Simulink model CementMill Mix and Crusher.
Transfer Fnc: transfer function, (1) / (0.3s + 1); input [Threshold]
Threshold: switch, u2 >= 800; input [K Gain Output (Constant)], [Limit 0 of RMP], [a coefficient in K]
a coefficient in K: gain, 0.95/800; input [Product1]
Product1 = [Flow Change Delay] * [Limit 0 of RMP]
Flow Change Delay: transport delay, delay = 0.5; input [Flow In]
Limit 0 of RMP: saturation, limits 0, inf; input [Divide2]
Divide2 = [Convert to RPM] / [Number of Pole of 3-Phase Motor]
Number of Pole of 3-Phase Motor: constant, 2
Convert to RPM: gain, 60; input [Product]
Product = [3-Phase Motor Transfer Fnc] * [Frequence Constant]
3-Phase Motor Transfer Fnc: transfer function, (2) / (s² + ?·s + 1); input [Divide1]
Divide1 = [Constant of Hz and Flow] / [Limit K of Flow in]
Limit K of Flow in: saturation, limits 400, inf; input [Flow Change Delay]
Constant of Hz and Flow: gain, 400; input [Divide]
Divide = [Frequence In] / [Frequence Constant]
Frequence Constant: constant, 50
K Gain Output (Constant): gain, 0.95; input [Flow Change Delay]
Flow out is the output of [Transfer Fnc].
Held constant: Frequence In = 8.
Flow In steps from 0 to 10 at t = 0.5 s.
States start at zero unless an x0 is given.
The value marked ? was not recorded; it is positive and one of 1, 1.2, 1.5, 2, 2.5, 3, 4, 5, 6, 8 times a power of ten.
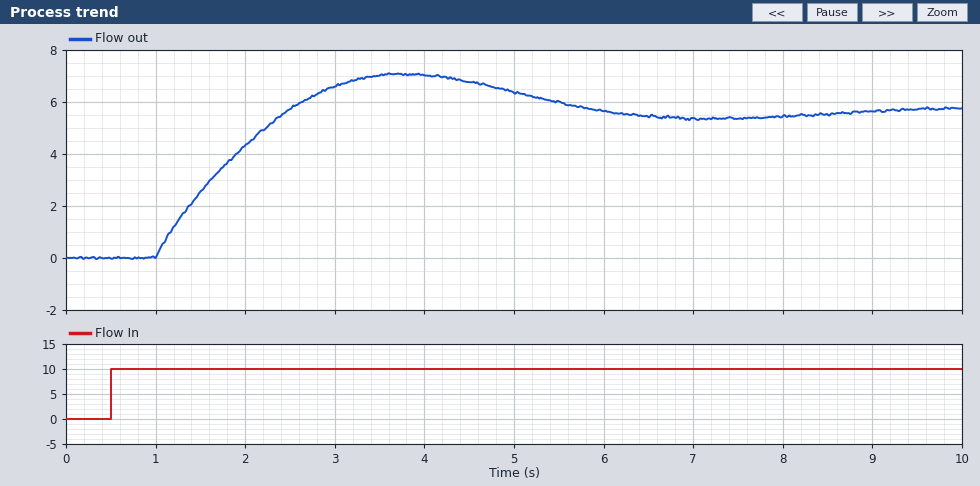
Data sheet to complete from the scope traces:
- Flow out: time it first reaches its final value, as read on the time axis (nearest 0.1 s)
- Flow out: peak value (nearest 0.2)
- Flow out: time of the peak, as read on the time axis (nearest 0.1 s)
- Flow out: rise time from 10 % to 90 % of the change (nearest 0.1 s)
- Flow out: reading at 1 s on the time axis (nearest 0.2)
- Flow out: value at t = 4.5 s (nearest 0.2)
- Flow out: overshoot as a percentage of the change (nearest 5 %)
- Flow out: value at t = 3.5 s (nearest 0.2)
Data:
2.5 s
7.0
3.8 s
1.2 s
0.0
6.8
25 %
7.0
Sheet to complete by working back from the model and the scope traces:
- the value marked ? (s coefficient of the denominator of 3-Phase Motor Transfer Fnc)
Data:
0.8
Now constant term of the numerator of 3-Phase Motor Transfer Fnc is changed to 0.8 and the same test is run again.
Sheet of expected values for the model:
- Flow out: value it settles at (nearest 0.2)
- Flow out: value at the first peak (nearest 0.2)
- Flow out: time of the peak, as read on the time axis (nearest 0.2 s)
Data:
2.2
2.8
3.8 s
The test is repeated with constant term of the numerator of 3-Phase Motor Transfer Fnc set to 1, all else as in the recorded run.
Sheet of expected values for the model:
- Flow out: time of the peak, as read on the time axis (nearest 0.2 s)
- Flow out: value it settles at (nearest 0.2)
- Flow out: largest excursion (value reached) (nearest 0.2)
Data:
3.8 s
2.8
3.6
